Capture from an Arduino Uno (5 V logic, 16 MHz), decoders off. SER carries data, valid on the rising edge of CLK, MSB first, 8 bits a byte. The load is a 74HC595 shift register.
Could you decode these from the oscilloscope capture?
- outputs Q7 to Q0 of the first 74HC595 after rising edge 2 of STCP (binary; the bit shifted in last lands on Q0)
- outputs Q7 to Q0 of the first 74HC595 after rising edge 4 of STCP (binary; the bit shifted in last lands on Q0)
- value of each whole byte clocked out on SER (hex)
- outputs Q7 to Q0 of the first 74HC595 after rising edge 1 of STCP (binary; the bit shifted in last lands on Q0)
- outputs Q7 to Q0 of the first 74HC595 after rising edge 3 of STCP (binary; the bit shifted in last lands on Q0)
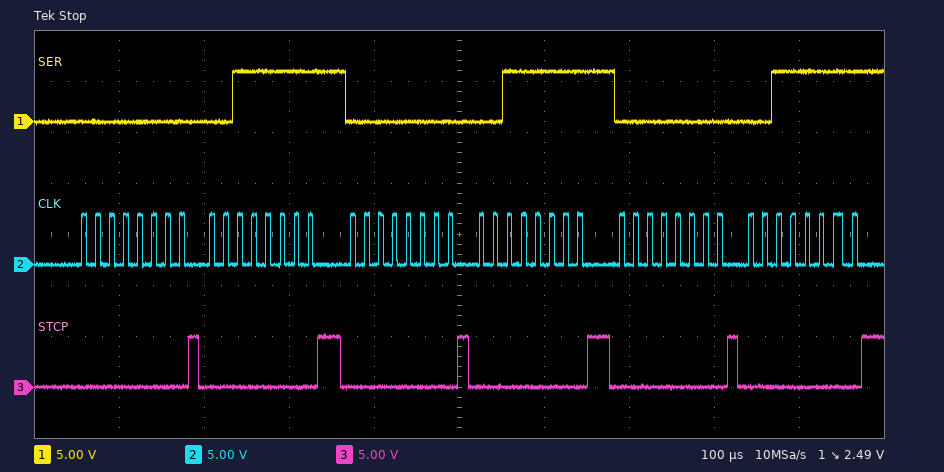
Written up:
00111111
00111111
0x00 0x3F 0x00 0x3F 0x00 0x3F
00000000
00000000
